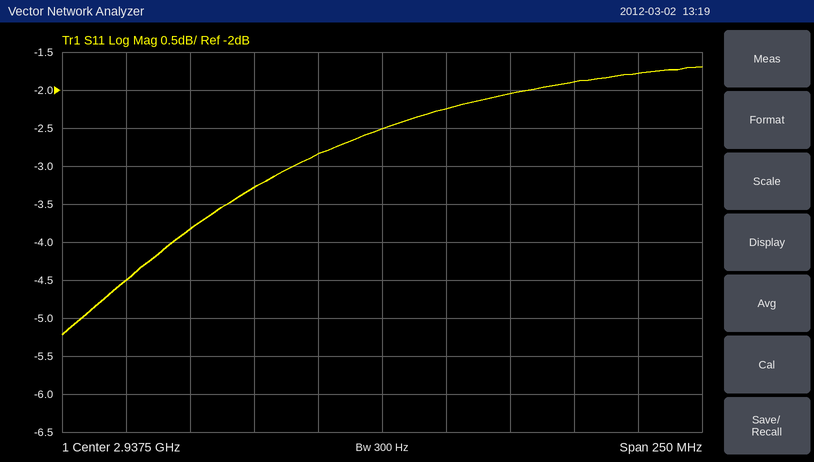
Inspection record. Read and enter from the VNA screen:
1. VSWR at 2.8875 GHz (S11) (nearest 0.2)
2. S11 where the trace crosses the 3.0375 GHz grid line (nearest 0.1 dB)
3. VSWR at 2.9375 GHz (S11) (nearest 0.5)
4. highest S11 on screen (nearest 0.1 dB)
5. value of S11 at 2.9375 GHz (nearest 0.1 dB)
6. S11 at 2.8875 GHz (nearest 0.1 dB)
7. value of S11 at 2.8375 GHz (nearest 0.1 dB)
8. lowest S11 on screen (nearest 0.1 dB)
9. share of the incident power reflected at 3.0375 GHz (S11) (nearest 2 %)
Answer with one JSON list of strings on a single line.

["5.4", "-1.8 dB", "7.0", "-1.7 dB", "-2.5 dB", "-3.3 dB", "-4.5 dB", "-5.2 dB", "66 %"]
